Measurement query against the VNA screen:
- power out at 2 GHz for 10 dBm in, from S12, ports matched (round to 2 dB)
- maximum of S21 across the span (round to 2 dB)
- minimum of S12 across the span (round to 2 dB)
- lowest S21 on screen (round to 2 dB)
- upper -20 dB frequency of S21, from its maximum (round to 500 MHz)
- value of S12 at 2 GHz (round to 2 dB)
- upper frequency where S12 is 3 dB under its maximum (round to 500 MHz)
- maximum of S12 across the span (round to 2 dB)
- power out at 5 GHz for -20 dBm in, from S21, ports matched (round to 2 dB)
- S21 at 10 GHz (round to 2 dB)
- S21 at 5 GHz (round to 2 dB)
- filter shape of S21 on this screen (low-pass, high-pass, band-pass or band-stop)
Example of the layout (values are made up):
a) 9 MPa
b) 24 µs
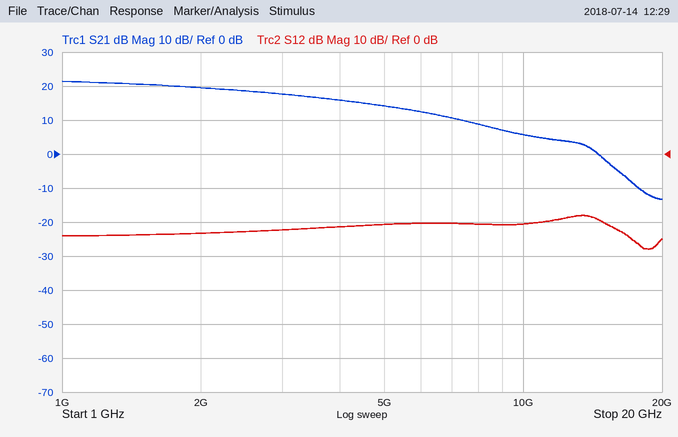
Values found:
a) -14 dBm
b) 22 dB
c) -28 dB
d) -14 dB
e) 14.0 GHz
f) -24 dB
g) 15.5 GHz
h) -18 dB
i) -6 dBm
j) 6 dB
k) 14 dB
l) low-pass
